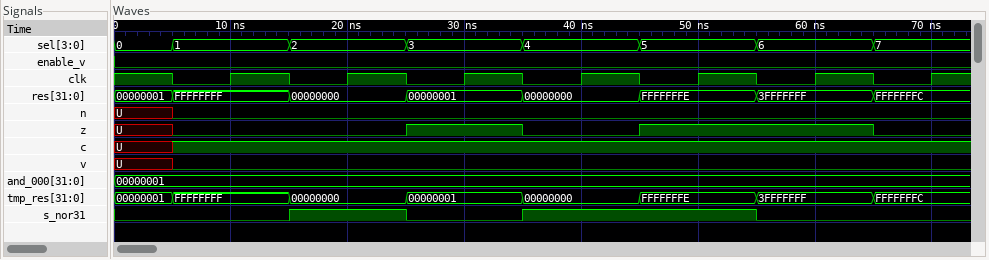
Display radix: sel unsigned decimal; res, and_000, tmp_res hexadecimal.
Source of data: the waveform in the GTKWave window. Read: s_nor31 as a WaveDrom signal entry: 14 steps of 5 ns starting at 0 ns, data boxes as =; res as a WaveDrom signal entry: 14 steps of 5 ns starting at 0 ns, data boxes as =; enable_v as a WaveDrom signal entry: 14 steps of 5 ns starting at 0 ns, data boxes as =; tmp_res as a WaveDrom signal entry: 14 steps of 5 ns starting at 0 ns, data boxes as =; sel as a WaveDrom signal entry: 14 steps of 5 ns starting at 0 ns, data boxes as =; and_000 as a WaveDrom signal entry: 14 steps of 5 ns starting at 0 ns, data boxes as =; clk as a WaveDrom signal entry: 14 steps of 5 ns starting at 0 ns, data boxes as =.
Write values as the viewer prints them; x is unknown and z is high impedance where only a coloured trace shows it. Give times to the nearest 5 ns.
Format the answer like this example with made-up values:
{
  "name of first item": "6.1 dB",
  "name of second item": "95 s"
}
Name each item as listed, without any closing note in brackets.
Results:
{
  "s_nor31 as a WaveDrom signal entry: 14 steps of 5 ns starting at 0 ns, data boxes as =": "{name: 's_nor31', wave: '0..1.0.1...0..'}",
  "res as a WaveDrom signal entry: 14 steps of 5 ns starting at 0 ns, data boxes as =": "{name: 'res', wave: '==.=.=.=.=.=.=', data: '00000001 FFFFFFFF 00000000 00000001 00000000 FFFFFFFE 3FFFFFFF FFFFFFFC'}",
  "enable_v as a WaveDrom signal entry: 14 steps of 5 ns starting at 0 ns, data boxes as =": "{name: 'enable_v', wave: '0.............'}",
  "tmp_res as a WaveDrom signal entry: 14 steps of 5 ns starting at 0 ns, data boxes as =": "{name: 'tmp_res', wave: '==.=.=.=.=.=.=', data: '00000001 FFFFFFFF 00000000 00000001 00000000 FFFFFFFE 3FFFFFFF FFFFFFFC'}",
  "sel as a WaveDrom signal entry: 14 steps of 5 ns starting at 0 ns, data boxes as =": "{name: 'sel', wave: '==.=.=.=.=.=.=', data: '0 1 2 3 4 5 6 7'}",
  "and_000 as a WaveDrom signal entry: 14 steps of 5 ns starting at 0 ns, data boxes as =": "{name: 'and_000', wave: '=.............', data: '00000001'}",
  "clk as a WaveDrom signal entry: 14 steps of 5 ns starting at 0 ns, data boxes as =": "{name: 'clk', wave: '10101010101010'}"
}
